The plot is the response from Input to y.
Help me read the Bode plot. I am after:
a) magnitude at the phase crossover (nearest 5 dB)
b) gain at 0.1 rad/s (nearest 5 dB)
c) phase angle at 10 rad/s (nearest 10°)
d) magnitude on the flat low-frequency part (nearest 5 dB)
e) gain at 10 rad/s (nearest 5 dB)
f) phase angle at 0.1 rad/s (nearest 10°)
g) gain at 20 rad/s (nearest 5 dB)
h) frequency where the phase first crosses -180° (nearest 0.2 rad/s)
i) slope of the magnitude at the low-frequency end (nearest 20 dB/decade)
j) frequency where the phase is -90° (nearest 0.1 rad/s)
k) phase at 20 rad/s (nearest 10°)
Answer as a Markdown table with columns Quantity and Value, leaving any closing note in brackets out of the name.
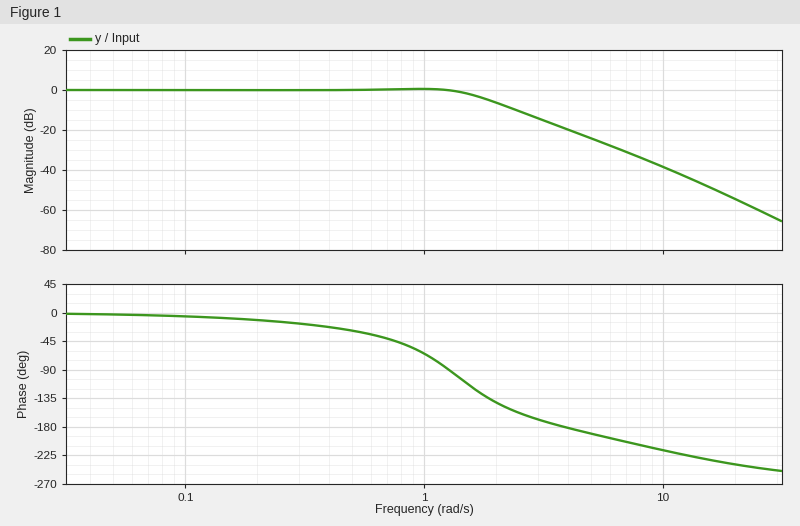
| Quantity | Value |
|---|---|
| magnitude at the phase crossover | -20 dB |
| gain at 0.1 rad/s | 0 dB |
| phase angle at 10 rad/s | -220° |
| magnitude on the flat low-frequency part | 0 dB |
| gain at 10 rad/s | -40 dB |
| phase angle at 0.1 rad/s | -10° |
| gain at 20 rad/s | -55 dB |
| frequency where the phase first crosses -180° | 3.8 rad/s |
| slope of the magnitude at the low-frequency end | 0 dB/decade |
| frequency where the phase is -90° | 1.3 rad/s |
| phase at 20 rad/s | -240° |
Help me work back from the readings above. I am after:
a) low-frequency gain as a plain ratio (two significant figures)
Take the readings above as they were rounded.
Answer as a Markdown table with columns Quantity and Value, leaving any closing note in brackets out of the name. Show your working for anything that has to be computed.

| Quantity | Value |
|---|---|
| low-frequency gain as a plain ratio | 10^(0 / 20) = 1.0 |
